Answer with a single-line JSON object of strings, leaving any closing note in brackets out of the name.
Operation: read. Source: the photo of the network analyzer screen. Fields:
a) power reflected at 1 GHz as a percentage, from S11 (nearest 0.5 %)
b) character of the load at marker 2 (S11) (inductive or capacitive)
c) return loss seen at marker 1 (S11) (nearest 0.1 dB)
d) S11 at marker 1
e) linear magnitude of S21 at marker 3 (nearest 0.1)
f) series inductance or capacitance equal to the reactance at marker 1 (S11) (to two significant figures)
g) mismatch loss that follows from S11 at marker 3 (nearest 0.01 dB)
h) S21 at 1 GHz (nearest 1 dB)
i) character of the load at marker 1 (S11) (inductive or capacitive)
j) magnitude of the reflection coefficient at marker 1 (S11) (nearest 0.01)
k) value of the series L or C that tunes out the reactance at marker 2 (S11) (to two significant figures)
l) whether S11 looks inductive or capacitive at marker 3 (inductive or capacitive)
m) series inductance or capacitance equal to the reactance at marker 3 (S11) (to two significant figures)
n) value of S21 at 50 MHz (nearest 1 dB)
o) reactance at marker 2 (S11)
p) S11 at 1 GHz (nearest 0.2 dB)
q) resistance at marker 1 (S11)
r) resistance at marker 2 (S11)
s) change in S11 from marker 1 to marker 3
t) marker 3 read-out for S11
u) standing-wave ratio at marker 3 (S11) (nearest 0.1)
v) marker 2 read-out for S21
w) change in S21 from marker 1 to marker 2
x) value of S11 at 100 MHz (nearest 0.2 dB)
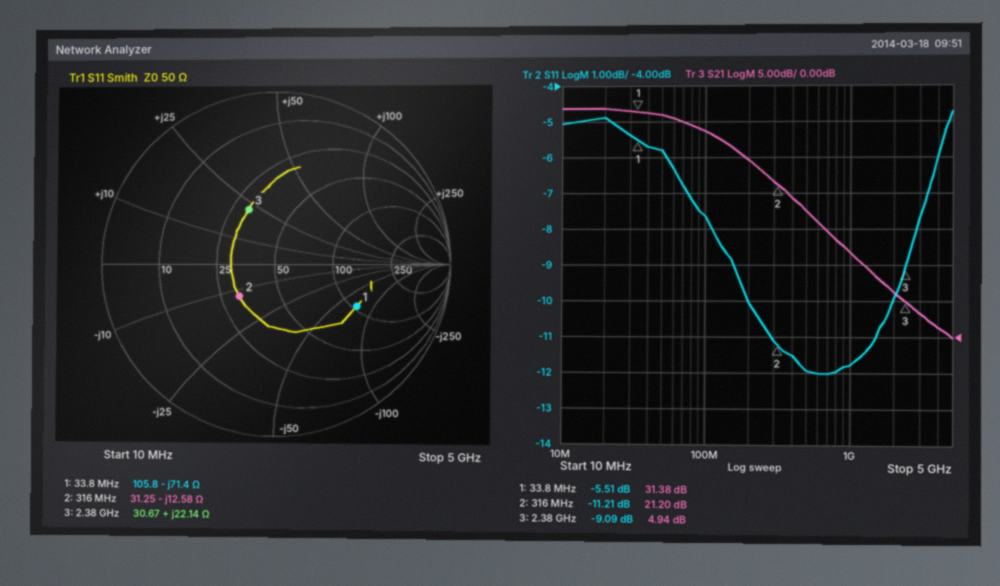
{"power reflected at 1 GHz as a percentage, from S11": "6.5 %", "character of the load at marker 2 (S11)": "capacitive", "return loss seen at marker 1 (S11)": "5.5 dB", "S11 at marker 1": "-5.51 dB", "linear magnitude of S21 at marker 3": "1.8", "series inductance or capacitance equal to the reactance at marker 1 (S11)": "66 pF", "mismatch loss that follows from S11 at marker 3": "0.57 dB", "S21 at 1 GHz": "12 dB", "character of the load at marker 1 (S11)": "capacitive", "magnitude of the reflection coefficient at marker 1 (S11)": "0.53", "value of the series L or C that tunes out the reactance at marker 2 (S11)": "6.3 nH", "whether S11 looks inductive or capacitive at marker 3": "inductive", "series inductance or capacitance equal to the reactance at marker 3 (S11)": "1.5 nH", "value of S21 at 50 MHz": "31 dB", "reactance at marker 2": "-12.58 Ω", "S11 at 1 GHz": "-11.8 dB", "resistance at marker 1": "105.8 Ω", "resistance at marker 2": "31.25 Ω", "change in S11 from marker 1 to marker 3": "-3.58 dB", "marker 3 read-out for S11": "-9.09 dB", "standing-wave ratio at marker 3 (S11)": "2.1", "marker 2 read-out for S21": "21.20 dB", "change in S21 from marker 1 to marker 2": "-10.18 dB", "value of S11 at 100 MHz": "-7.6 dB"}
